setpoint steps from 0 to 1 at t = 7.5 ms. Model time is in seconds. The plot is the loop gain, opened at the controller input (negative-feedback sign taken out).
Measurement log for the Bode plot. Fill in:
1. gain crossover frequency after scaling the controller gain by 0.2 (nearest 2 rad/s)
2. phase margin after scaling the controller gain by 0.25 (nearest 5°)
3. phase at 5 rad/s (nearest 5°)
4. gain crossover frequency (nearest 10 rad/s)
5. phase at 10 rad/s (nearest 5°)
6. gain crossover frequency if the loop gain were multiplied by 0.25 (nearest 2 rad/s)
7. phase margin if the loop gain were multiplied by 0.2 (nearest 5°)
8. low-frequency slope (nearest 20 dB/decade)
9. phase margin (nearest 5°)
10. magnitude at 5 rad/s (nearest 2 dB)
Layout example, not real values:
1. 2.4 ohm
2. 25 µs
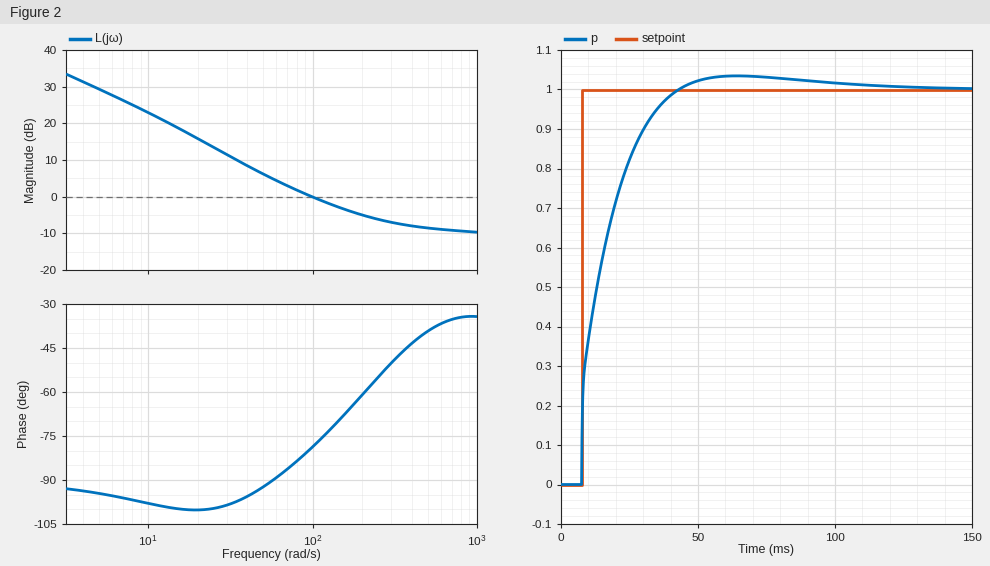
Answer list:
1. 24 rad/s
2. 80°
3. -95°
4. 100 rad/s
5. -100°
6. 28 rad/s
7. 80°
8. -20 dB/decade
9. 100°
10. 30 dB
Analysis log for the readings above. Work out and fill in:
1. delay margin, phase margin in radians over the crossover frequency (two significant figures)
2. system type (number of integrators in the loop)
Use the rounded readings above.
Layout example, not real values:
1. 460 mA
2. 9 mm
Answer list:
1. 0.017 s
2. 1
